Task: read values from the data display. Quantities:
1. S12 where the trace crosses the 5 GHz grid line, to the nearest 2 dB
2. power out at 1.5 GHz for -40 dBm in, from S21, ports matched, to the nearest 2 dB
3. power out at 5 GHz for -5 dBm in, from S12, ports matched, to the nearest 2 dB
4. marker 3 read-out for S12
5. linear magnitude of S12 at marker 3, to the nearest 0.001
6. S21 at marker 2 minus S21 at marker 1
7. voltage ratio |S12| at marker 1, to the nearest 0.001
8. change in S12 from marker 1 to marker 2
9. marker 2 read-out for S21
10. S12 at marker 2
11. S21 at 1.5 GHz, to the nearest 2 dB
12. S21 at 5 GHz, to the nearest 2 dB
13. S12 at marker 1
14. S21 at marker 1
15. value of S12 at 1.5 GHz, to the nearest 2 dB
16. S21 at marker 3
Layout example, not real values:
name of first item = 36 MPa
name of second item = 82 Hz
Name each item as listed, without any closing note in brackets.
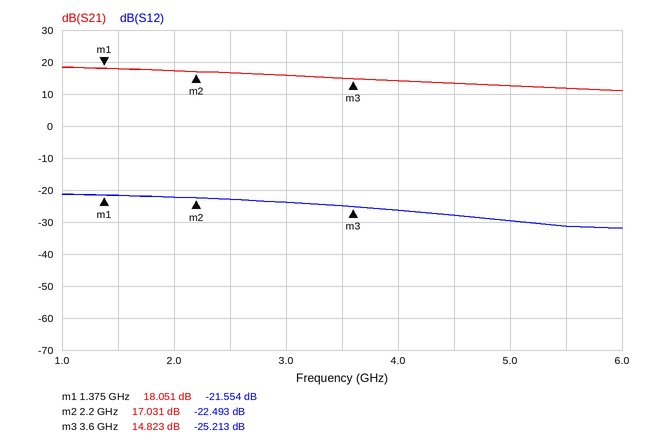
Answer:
S12 where the trace crosses the 5 GHz grid line, to the nearest 2 dB = -30 dB
power out at 1.5 GHz for -40 dBm in, from S21, ports matched, to the nearest 2 dB = -22 dBm
power out at 5 GHz for -5 dBm in, from S12, ports matched, to the nearest 2 dB = -34 dBm
marker 3 read-out for S12 = -25.213 dB
linear magnitude of S12 at marker 3, to the nearest 0.001 = 0.055
S21 at marker 2 minus S21 at marker 1 = -1.020 dB
voltage ratio |S12| at marker 1, to the nearest 0.001 = 0.084
change in S12 from marker 1 to marker 2 = -0.939 dB
marker 2 read-out for S21 = 17.031 dB
S12 at marker 2 = -22.493 dB
S21 at 1.5 GHz, to the nearest 2 dB = 18 dB
S21 at 5 GHz, to the nearest 2 dB = 12 dB
S12 at marker 1 = -21.554 dB
S21 at marker 1 = 18.051 dB
value of S12 at 1.5 GHz, to the nearest 2 dB = -22 dB
S21 at marker 3 = 14.823 dB
